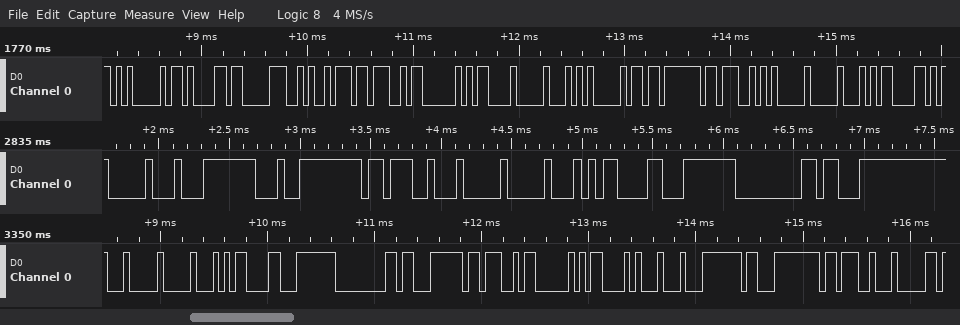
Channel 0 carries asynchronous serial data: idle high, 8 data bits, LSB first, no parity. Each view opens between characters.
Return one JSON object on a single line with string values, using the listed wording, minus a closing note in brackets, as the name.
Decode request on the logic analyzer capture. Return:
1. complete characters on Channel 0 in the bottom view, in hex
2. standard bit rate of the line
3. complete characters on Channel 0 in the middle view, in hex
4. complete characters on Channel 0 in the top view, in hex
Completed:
{"complete characters on Channel 0 in the bottom view, in hex": "04, 10, 0D, FC, 00, E3, 3B, 03, 0D, 11, FC, E3, 3B, 04", "standard bit rate of the line": "19200 baud", "complete characters on Channel 0 in the middle view, in hex": "10, FC, E4, 3B, 04, 10, 0D, FC, 00, E3", "complete characters on Channel 0 in the top view, in hex": "05, 0B, 83, 4A, 3B, 03, 0D, 10, 05, DB, 3B, 05, 10, 0D"}
